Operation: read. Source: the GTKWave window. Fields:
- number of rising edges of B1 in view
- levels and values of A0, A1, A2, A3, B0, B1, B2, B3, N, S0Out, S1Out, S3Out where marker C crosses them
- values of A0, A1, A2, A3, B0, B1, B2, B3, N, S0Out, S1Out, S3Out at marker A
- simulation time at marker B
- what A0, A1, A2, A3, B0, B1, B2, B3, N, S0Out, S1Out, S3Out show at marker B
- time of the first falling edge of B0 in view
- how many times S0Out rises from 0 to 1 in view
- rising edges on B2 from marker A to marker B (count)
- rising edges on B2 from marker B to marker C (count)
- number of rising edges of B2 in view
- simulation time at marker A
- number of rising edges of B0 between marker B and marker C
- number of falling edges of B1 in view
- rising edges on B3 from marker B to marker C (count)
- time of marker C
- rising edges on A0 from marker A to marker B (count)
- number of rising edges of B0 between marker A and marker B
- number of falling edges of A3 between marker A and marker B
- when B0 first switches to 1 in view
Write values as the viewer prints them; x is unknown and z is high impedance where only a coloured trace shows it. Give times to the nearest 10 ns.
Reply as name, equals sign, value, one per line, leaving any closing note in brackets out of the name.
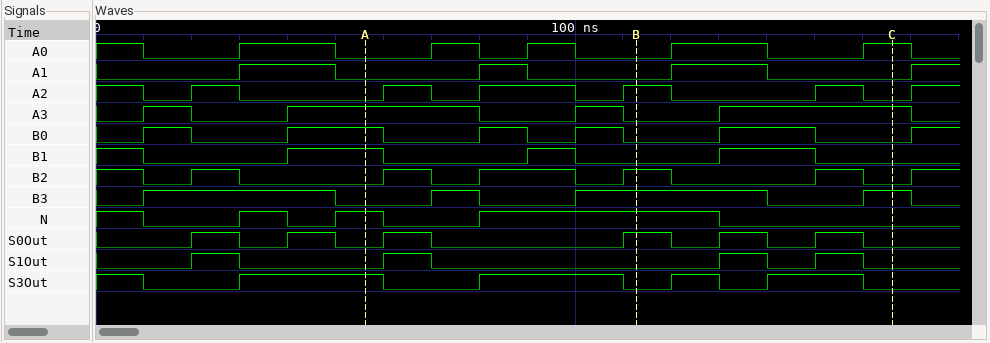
number of rising edges of B1 in view = 3
levels and values of A0, A1, A2, A3, B0, B1, B2, B3, N, S0Out, S1Out, S3Out where marker C crosses them = A0=1, A1=0, A2=0, A3=1, B0=0, B1=0, B2=0, B3=1, N=0, S0Out=0, S1Out=0, S3Out=0
values of A0, A1, A2, A3, B0, B1, B2, B3, N, S0Out, S1Out, S3Out at marker A = A0=0, A1=0, A2=0, A3=1, B0=1, B1=1, B2=0, B3=0, N=1, S0Out=0, S1Out=0, S3Out=1
simulation time at marker B = 110 ns
what A0, A1, A2, A3, B0, B1, B2, B3, N, S0Out, S1Out, S3Out show at marker B = A0=0, A1=0, A2=1, A3=0, B0=0, B1=0, B2=1, B3=1, N=1, S0Out=1, S1Out=0, S3Out=0
time of the first falling edge of B0 in view = 20 ns
how many times S0Out rises from 0 to 1 in view = 6
rising edges on B2 from marker A to marker B = 3
rising edges on B2 from marker B to marker C = 1
number of rising edges of B2 in view = 6
simulation time at marker A = 60 ns
number of rising edges of B0 between marker B and marker C = 1
number of falling edges of B1 in view = 4
rising edges on B3 from marker B to marker C = 1
time of marker C = 170 ns
rising edges on A0 from marker A to marker B = 2
number of rising edges of B0 between marker A and marker B = 2
number of falling edges of A3 between marker A and marker B = 2
when B0 first switches to 1 in view = 10 ns
